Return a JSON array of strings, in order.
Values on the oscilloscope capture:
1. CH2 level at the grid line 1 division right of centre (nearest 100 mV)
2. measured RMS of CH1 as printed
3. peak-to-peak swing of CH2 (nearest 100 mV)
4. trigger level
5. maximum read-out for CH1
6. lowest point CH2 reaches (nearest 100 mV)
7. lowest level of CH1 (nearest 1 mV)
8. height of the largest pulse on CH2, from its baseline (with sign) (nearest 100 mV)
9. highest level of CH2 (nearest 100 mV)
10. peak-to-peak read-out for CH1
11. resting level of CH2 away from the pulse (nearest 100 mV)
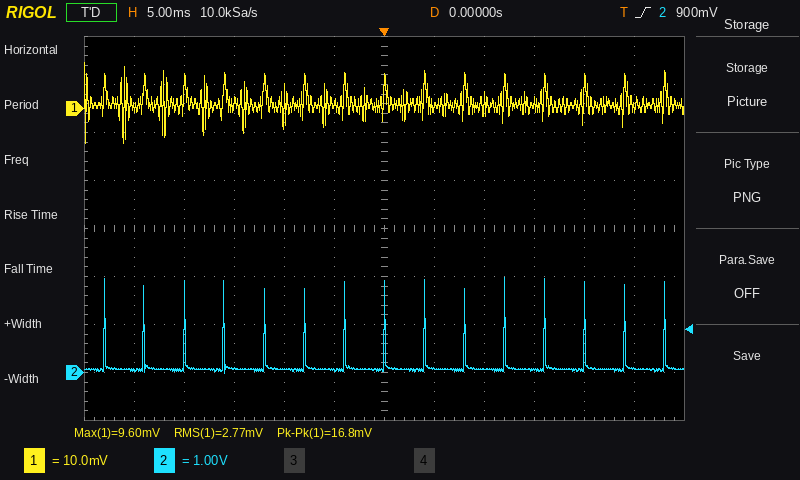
["100 mV", "2.77 mV", "2.0 V", "900 mV", "9.60 mV", "0.0 V", "-7 mV", "+1.9 V", "2.0 V", "16.8 mV", "100 mV"]
